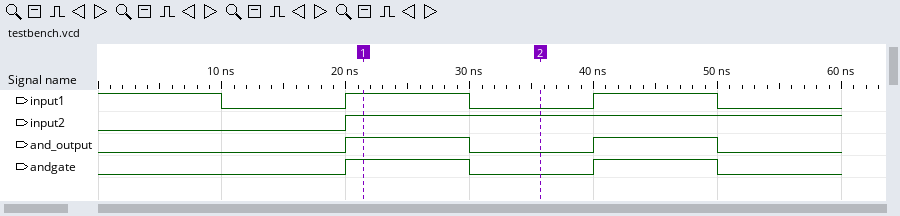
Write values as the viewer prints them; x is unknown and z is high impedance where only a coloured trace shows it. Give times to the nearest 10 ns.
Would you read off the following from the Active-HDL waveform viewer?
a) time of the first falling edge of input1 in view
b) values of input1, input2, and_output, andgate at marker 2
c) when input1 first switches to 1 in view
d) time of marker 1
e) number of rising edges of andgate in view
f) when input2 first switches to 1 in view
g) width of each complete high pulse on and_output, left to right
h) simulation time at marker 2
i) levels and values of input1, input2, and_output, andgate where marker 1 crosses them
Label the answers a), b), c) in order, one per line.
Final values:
a) 10 ns
b) input1=0, input2=1, and_output=0, andgate=0
c) 20 ns
d) 20 ns
e) 2
f) 20 ns
g) 10 ns, 10 ns
h) 40 ns
i) input1=1, input2=1, and_output=1, andgate=1
